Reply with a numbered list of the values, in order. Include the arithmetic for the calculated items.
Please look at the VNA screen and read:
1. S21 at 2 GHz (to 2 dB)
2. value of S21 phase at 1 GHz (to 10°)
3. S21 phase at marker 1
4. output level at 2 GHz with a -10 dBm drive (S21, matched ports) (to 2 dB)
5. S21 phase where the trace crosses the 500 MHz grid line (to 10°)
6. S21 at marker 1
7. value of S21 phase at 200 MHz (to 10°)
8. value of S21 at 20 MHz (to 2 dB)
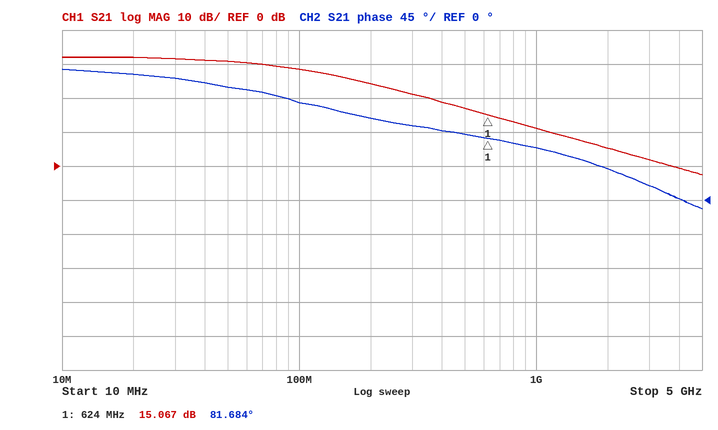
1. 6 dB
2. 70°
3. 81.684°
4. -10 dBm + (6 dB) = -4 dBm
5. 90°
6. 15.067 dB
7. 110°
8. 32 dB
